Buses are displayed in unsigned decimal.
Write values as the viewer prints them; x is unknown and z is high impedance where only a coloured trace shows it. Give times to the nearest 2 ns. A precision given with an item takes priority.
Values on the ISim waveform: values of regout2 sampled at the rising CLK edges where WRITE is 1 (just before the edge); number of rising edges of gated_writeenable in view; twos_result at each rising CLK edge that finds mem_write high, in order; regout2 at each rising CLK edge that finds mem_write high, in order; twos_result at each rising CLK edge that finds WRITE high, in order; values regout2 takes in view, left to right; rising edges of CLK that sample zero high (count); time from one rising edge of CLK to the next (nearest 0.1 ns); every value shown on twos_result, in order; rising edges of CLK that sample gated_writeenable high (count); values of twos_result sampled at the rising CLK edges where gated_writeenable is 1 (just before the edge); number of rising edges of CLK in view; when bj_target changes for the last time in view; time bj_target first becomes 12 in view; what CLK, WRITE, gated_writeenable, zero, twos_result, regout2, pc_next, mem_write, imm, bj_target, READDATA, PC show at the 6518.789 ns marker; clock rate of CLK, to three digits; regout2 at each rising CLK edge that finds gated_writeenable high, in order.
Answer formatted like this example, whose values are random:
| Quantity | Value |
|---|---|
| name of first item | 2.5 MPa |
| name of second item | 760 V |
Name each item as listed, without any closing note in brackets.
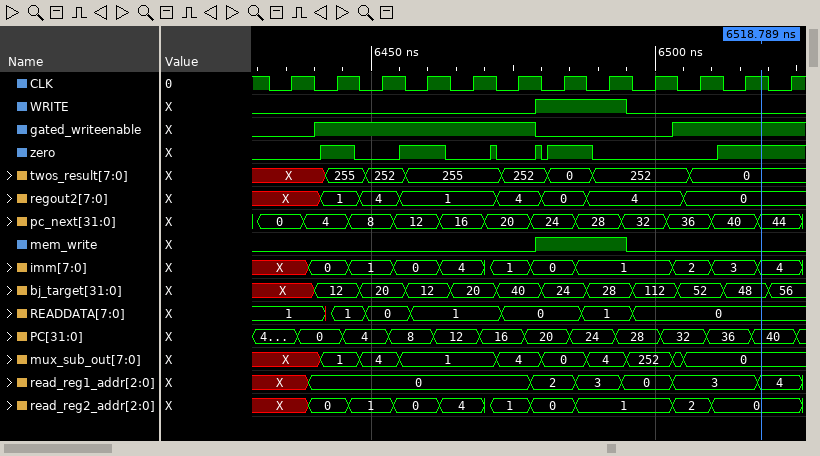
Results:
| Quantity | Value |
|---|---|
| values of regout2 sampled at the rising CLK edges where WRITE is 1 | 0, 4 |
| number of rising edges of gated_writeenable in view | 2 |
| twos_result at each rising CLK edge that finds mem_write high, in order | 0, 252 |
| regout2 at each rising CLK edge that finds mem_write high, in order | 0, 4 |
| twos_result at each rising CLK edge that finds WRITE high, in order | 0, 252 |
| values regout2 takes in view, left to right | X, 1, 4, 1, 4, 0, 4, 0 |
| rising edges of CLK that sample zero high | 5 |
| time from one rising edge of CLK to the next | 8 ns |
| every value shown on twos_result, in order | X, 255, 252, 255, 252, 0, 252, 0 |
| rising edges of CLK that sample gated_writeenable high | 8 |
| values of twos_result sampled at the rising CLK edges where gated_writeenable is 1 | 255, 252, 255, 255, 252, 0, 0, 0 |
| number of rising edges of CLK in view | 12 |
| when bj_target changes for the last time in view | 6520 ns |
| time bj_target first becomes 12 in view | 6440 ns |
| what CLK, WRITE, gated_writeenable, zero, twos_result, regout2, pc_next, mem_write, imm, bj_target, READDATA, PC show at the 6518.789 ns marker | CLK=1, WRITE=0, gated_writeenable=1, zero=1, twos_result=0, regout2=0, pc_next=44, mem_write=0, imm=4, bj_target=48, READDATA=0, PC=40 |
| clock rate of CLK, to three digits | 125 MHz |
| regout2 at each rising CLK edge that finds gated_writeenable high, in order | 1, 4, 1, 1, 4, 0, 0, 0 |
